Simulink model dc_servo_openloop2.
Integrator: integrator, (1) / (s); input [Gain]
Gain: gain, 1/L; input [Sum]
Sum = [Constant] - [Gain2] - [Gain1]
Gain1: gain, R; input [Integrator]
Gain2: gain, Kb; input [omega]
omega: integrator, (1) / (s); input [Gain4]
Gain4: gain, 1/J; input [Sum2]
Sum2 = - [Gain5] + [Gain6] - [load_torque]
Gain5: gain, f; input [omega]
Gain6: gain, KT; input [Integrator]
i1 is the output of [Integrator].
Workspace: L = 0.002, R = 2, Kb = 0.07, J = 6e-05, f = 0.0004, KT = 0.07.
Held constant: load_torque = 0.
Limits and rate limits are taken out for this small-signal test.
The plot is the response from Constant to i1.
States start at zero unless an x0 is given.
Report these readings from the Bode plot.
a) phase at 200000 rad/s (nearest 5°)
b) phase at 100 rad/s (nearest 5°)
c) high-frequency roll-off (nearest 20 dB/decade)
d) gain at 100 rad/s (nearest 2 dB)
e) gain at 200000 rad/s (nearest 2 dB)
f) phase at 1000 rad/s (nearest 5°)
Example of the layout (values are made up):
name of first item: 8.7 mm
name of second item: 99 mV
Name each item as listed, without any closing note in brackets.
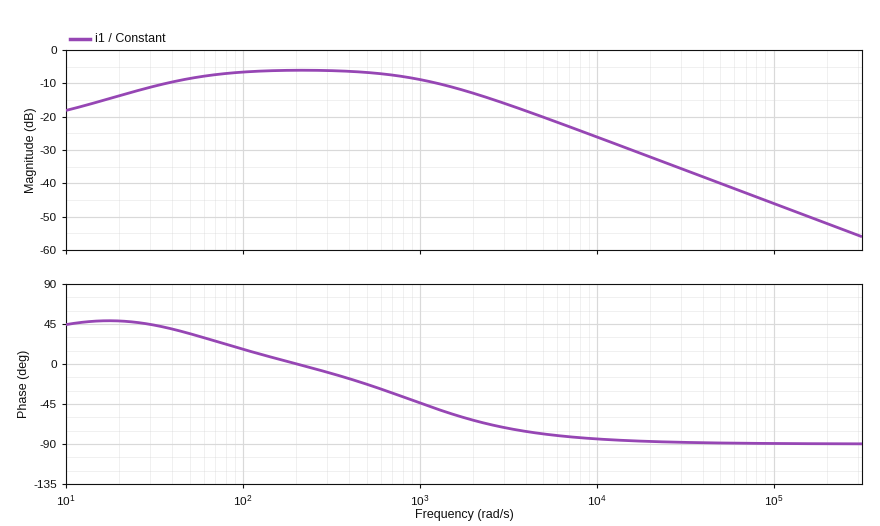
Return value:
phase at 200000 rad/s: -90°
phase at 100 rad/s: 15°
high-frequency roll-off: -20 dB/decade
gain at 100 rad/s: -6 dB
gain at 200000 rad/s: -52 dB
phase at 1000 rad/s: -45°
